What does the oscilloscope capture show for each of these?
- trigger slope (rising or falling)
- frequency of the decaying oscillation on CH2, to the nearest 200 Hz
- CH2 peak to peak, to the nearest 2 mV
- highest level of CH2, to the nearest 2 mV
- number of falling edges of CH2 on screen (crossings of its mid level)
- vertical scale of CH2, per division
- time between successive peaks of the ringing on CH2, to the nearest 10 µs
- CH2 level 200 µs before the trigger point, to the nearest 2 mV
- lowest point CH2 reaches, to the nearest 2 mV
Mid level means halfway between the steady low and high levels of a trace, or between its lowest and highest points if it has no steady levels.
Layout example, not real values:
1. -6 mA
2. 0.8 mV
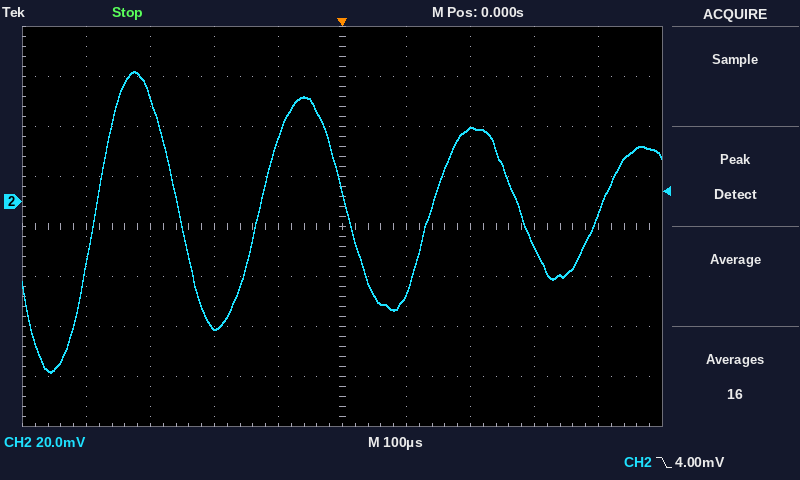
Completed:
1. falling
2. 3.8 kHz
3. 120 mV
4. 52 mV
5. 3
6. 20 mV
7. 260 µs
8. -50 mV
9. -68 mV
